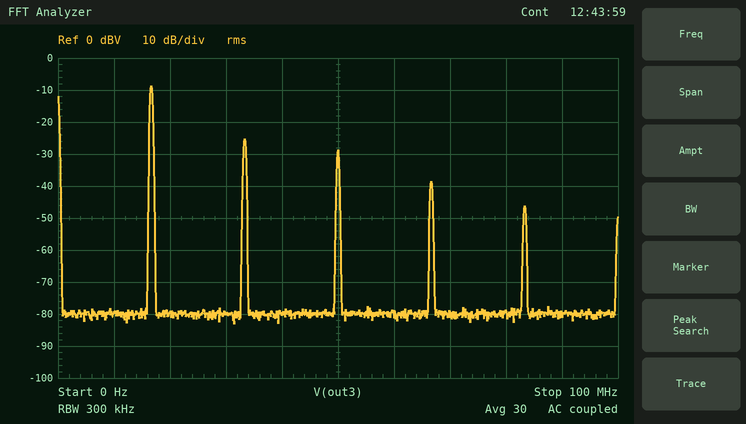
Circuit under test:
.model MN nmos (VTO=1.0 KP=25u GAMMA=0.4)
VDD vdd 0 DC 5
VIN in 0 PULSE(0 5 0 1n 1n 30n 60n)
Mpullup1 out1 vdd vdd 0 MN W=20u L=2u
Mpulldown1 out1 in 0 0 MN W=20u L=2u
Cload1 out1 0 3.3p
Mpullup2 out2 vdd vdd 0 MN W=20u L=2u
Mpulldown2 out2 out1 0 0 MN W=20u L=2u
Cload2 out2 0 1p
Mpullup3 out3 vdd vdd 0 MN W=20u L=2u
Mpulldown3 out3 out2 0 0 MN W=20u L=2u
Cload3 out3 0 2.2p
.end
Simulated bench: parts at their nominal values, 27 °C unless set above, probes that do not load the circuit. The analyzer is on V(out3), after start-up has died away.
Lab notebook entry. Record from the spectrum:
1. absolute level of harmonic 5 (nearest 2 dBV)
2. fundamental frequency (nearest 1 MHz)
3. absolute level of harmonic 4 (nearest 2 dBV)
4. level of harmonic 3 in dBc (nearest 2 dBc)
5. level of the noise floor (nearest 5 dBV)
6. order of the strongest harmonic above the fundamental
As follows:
-46 dBV
17 MHz
-38 dBV
-20 dBc
-80 dBV
2
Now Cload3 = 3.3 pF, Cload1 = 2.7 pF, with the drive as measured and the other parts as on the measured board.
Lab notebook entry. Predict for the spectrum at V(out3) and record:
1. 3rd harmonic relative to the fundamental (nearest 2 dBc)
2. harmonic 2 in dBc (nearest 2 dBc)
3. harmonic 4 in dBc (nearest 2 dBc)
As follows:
-22 dBc
-20 dBc
-34 dBc
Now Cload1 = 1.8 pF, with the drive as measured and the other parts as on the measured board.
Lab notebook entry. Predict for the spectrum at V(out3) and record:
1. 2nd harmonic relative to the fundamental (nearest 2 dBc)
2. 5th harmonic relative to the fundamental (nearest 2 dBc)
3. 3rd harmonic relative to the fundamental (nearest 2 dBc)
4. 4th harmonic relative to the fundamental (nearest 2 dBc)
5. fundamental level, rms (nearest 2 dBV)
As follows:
-20 dBc
-34 dBc
-18 dBc
-32 dBc
-8 dBV
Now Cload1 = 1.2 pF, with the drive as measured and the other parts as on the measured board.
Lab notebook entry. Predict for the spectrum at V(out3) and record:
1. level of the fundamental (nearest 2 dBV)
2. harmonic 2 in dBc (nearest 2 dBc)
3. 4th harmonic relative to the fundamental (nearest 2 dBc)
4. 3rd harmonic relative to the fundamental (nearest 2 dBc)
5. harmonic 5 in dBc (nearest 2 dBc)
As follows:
-6 dBV
-22 dBc
-34 dBc
-18 dBc
-32 dBc
